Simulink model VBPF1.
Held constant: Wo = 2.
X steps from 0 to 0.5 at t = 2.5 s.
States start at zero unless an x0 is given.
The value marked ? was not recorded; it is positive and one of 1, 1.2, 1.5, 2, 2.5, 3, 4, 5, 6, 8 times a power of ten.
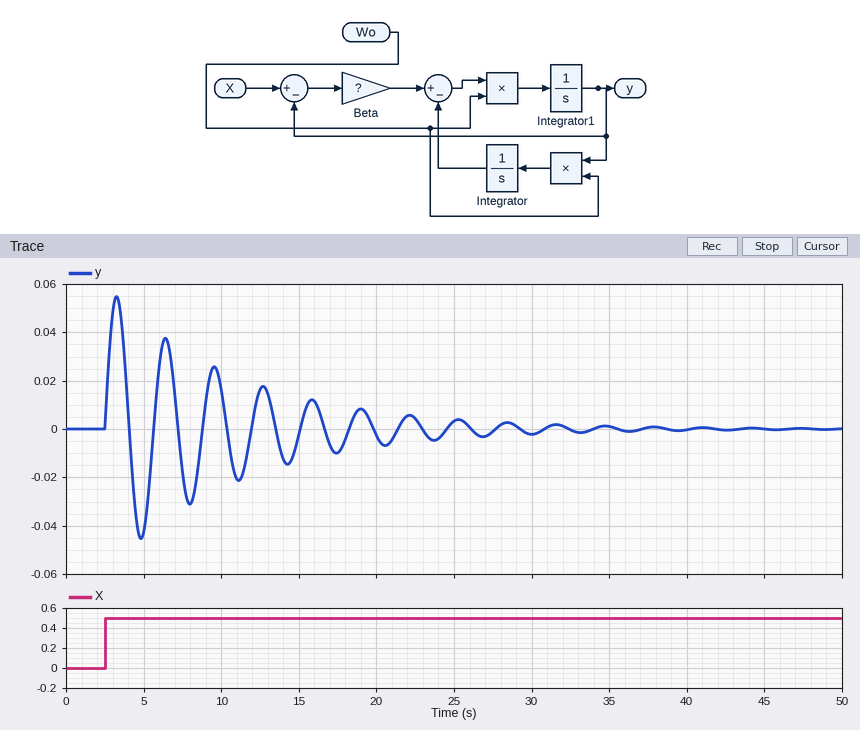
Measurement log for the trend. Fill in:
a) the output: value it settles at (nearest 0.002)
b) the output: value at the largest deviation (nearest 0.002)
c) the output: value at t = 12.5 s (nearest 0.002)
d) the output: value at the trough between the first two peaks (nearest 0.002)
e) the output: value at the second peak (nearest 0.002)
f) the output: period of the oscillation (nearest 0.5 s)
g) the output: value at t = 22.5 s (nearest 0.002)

0.000
0.054
0.016
-0.046
0.038
3.0 s
0.004
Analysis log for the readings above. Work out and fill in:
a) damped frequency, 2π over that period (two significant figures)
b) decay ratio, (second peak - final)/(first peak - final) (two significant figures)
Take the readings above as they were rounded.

2.1 rad/s
0.70
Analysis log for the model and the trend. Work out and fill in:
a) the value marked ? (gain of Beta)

0.12
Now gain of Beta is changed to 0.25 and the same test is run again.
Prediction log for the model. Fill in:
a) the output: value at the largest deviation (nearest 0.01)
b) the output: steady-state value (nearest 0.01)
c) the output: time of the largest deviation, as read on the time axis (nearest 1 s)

0.10
0.00
3 s
